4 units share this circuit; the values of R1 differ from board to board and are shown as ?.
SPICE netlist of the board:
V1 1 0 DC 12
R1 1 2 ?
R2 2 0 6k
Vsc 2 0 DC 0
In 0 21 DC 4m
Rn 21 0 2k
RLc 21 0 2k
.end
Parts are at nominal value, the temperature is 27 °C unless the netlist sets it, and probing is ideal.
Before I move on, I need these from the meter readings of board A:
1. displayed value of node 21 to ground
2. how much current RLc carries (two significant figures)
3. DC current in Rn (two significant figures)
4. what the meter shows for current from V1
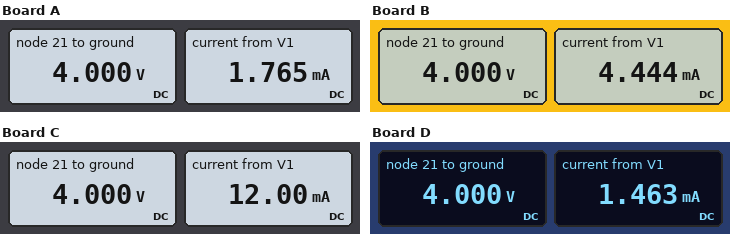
4.000 V
2.0 mA
2.0 mA
1.765 mA
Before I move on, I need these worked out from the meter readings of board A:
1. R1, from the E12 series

6.8 kΩ
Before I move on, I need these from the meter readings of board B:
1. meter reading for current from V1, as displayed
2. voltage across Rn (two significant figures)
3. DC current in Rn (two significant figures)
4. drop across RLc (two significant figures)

4.444 mA
4.0 V
2.0 mA
4.0 V
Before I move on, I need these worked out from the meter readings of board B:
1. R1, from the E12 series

2.7 kΩ
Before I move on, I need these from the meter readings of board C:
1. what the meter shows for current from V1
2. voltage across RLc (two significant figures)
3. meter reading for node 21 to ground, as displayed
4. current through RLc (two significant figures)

12.00 mA
4.0 V
4.000 V
2.0 mA
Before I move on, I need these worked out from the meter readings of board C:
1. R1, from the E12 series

1 kΩ
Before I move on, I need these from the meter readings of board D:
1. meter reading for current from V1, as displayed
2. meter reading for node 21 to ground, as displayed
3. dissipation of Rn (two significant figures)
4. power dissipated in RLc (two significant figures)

1.463 mA
4.000 V
8.0 mW
8.0 mW
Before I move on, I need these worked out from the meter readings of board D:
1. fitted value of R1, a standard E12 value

8.2 kΩ
